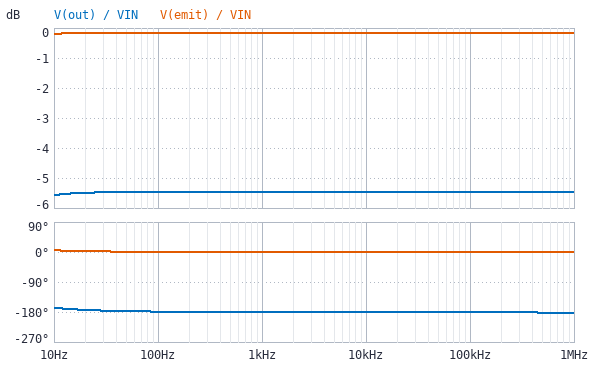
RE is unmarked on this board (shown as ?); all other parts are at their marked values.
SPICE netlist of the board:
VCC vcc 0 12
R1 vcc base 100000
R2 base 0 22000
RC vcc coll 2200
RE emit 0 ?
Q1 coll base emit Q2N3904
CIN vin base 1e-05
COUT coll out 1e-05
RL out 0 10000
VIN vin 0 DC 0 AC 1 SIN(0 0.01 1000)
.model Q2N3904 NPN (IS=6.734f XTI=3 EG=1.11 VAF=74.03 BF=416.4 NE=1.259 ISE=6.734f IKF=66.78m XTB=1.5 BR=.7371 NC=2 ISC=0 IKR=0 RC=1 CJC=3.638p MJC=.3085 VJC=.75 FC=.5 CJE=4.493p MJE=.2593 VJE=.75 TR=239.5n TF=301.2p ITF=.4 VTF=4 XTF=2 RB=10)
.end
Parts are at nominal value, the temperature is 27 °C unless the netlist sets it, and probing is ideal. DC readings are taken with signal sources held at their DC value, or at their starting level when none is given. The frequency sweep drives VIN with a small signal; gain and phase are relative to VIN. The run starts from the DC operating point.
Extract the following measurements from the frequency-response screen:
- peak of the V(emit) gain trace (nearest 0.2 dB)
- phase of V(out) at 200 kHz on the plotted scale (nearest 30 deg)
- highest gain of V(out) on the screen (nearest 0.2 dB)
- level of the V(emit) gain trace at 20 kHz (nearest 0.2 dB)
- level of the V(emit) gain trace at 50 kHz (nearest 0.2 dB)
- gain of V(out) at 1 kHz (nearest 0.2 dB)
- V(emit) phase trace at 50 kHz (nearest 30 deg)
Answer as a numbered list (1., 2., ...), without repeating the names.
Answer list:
1. -0.2 dB
2. -180 deg
3. -5.4 dB
4. -0.2 dB
5. -0.2 dB
6. -5.4 dB
7. 0 deg
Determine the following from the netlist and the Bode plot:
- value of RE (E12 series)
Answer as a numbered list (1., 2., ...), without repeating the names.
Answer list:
1. 3.3 kΩ
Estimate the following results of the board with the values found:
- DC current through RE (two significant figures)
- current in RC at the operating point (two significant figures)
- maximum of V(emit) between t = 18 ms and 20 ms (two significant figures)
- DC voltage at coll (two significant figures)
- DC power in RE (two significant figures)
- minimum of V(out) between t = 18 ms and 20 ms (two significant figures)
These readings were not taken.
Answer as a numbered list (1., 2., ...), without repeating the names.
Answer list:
1. 440 µA
2. 440 µA
3. 1.5 V
4. 11 V
5. 650 µW
6. -5.3 mV
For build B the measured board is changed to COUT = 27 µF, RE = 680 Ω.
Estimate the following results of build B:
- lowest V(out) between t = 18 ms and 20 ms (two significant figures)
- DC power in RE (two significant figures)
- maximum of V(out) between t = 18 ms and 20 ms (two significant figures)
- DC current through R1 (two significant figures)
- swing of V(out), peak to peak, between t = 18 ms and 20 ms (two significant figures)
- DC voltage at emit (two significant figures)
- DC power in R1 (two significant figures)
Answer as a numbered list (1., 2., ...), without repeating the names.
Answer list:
1. -26 mV
2. 2.4 mW
3. 26 mV
4. 100 µA
5. 52 mV
6. 1.3 V
7. 1.0 mW
